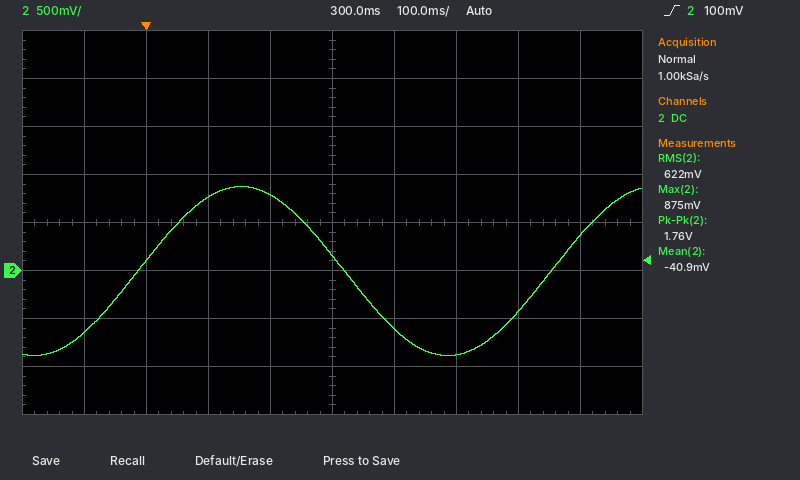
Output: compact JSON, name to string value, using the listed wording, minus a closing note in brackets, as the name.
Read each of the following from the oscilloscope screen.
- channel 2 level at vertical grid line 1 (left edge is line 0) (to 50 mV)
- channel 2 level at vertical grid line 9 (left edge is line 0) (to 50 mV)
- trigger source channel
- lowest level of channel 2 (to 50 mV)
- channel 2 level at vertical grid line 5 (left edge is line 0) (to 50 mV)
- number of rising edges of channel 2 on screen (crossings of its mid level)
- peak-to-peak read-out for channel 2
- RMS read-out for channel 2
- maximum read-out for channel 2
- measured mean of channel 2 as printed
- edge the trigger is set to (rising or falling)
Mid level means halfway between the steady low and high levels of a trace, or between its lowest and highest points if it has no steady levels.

{"channel 2 level at vertical grid line 1 (left edge is line 0)": "-650 mV", "channel 2 level at vertical grid line 9 (left edge is line 0)": "350 mV", "trigger source channel": "channel 2", "lowest level of channel 2": "-900 mV", "channel 2 level at vertical grid line 5 (left edge is line 0)": "150 mV", "number of rising edges of channel 2 on screen": "2", "peak-to-peak read-out for channel 2": "1.76 V", "RMS read-out for channel 2": "622 mV", "maximum read-out for channel 2": "875 mV", "measured mean of channel 2 as printed": "-40.9 mV", "edge the trigger is set to": "rising"}
